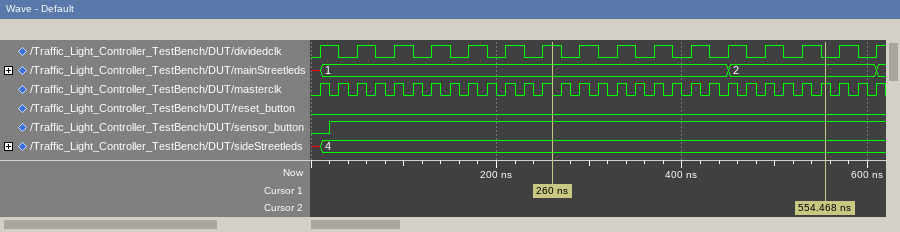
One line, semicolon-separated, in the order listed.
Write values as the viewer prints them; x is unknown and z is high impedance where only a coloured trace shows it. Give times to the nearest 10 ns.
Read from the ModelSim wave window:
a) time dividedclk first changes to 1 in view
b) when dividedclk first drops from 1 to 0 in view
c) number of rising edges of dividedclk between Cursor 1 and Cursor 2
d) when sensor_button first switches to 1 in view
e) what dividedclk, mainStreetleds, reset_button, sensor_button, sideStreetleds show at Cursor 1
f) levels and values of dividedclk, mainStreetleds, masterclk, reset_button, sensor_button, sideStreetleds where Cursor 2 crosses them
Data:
10 ns; 30 ns; 7; 20 ns; dividedclk=1, mainStreetleds=1, reset_button=0, sensor_button=1, sideStreetleds=4; dividedclk=0, mainStreetleds=2, masterclk=1, reset_button=0, sensor_button=1, sideStreetleds=4
